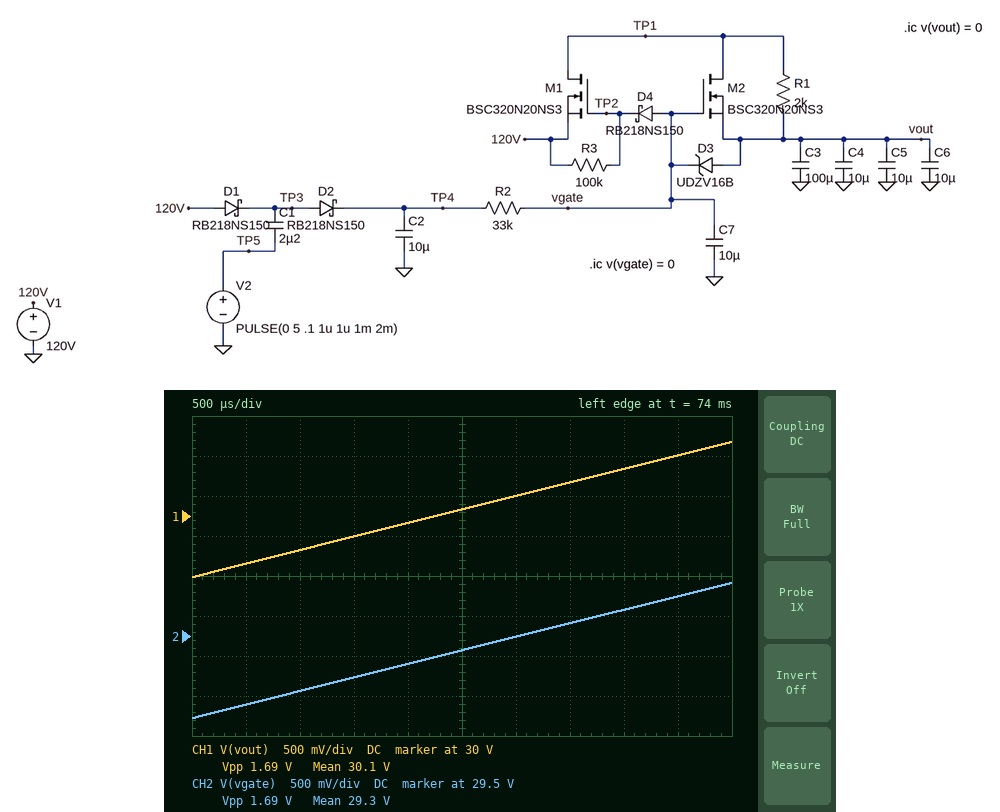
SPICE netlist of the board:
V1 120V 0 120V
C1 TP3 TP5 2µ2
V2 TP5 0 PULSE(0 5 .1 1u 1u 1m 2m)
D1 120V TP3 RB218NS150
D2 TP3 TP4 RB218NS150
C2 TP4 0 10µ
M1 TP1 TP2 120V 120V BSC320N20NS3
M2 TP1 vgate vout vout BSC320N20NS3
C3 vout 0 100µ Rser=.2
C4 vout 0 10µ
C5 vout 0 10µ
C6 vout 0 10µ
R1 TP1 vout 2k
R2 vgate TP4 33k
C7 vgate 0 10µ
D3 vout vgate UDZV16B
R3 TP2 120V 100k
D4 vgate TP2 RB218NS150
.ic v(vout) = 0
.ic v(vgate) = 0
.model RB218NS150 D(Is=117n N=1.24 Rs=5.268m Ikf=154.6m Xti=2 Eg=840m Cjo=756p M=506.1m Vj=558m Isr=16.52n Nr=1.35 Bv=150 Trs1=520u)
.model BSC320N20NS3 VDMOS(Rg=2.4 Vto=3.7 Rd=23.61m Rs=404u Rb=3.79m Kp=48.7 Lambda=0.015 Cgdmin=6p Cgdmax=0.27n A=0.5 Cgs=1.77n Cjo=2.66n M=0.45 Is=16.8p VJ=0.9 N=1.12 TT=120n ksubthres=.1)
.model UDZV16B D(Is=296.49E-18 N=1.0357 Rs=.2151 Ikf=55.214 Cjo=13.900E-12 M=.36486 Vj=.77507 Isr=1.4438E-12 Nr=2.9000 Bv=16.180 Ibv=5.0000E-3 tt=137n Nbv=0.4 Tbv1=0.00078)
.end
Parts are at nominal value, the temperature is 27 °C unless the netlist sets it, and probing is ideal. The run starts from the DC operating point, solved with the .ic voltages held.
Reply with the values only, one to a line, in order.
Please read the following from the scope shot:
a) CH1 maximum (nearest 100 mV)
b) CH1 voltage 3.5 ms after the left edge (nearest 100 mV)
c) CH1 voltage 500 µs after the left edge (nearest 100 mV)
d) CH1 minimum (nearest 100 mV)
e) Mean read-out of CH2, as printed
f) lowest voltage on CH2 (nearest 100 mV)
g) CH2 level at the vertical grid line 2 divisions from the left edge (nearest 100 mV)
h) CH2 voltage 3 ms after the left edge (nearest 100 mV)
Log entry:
30.9 V
30.4 V
29.4 V
29.2 V
29.3 V
28.5 V
28.8 V
29.5 V
